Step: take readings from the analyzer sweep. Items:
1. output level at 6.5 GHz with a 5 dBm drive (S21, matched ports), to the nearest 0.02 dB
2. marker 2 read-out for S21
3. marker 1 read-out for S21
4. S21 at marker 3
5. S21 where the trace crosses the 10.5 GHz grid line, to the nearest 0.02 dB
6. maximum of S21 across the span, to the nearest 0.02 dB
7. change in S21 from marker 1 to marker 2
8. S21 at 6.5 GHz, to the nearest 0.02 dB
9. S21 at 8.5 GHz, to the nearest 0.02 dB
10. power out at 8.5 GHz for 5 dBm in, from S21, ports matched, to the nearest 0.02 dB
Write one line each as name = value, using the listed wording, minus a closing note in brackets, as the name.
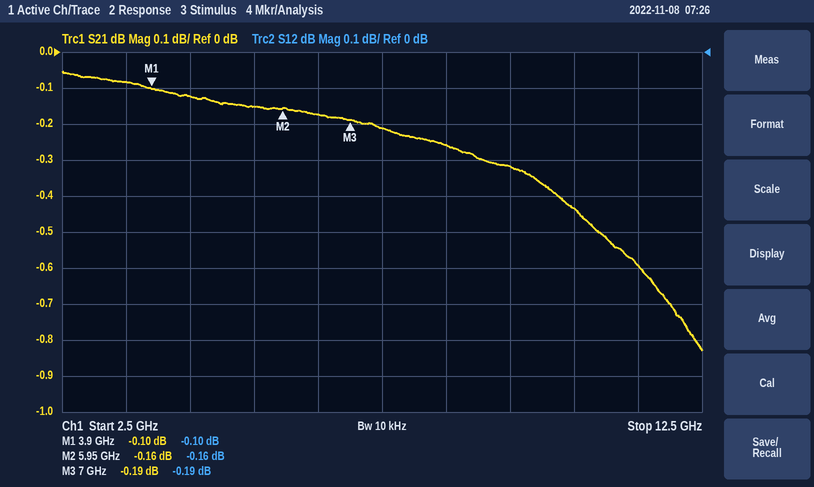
output level at 6.5 GHz with a 5 dBm drive (S21, matched ports), to the nearest 0.02 dB = 4.82 dBm
marker 2 read-out for S21 = -0.16 dB
marker 1 read-out for S21 = -0.10 dB
S21 at marker 3 = -0.19 dB
S21 where the trace crosses the 10.5 GHz grid line, to the nearest 0.02 dB = -0.44 dB
maximum of S21 across the span, to the nearest 0.02 dB = -0.06 dB
change in S21 from marker 1 to marker 2 = -0.06 dB
S21 at 6.5 GHz, to the nearest 0.02 dB = -0.18 dB
S21 at 8.5 GHz, to the nearest 0.02 dB = -0.26 dB
power out at 8.5 GHz for 5 dBm in, from S21, ports matched, to the nearest 0.02 dB = 4.74 dBm
